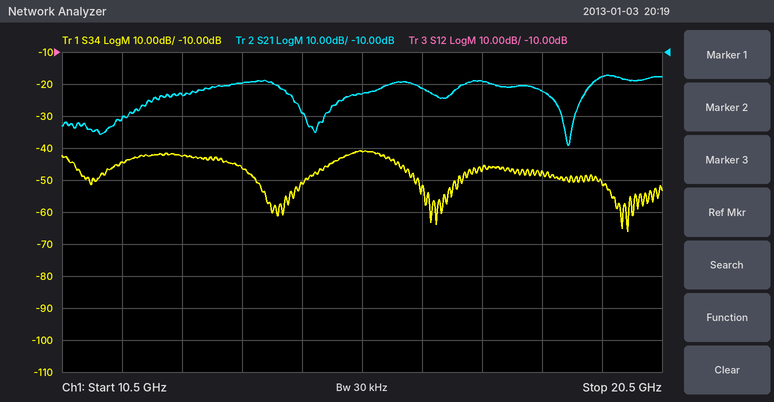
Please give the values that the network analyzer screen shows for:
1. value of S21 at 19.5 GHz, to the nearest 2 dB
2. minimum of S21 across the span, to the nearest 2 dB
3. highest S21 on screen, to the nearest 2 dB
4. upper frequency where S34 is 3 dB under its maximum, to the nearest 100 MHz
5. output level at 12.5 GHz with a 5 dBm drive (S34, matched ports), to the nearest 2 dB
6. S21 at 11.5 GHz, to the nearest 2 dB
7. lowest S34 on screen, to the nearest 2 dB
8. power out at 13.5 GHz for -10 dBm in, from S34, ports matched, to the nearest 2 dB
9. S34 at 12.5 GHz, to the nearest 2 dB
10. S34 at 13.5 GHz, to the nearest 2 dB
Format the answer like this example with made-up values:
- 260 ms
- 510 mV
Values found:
- -18 dB
- -40 dB
- -18 dB
- 16.0 GHz
- -38 dBm
- -30 dB
- -66 dB
- -56 dBm
- -42 dB
- -46 dB
